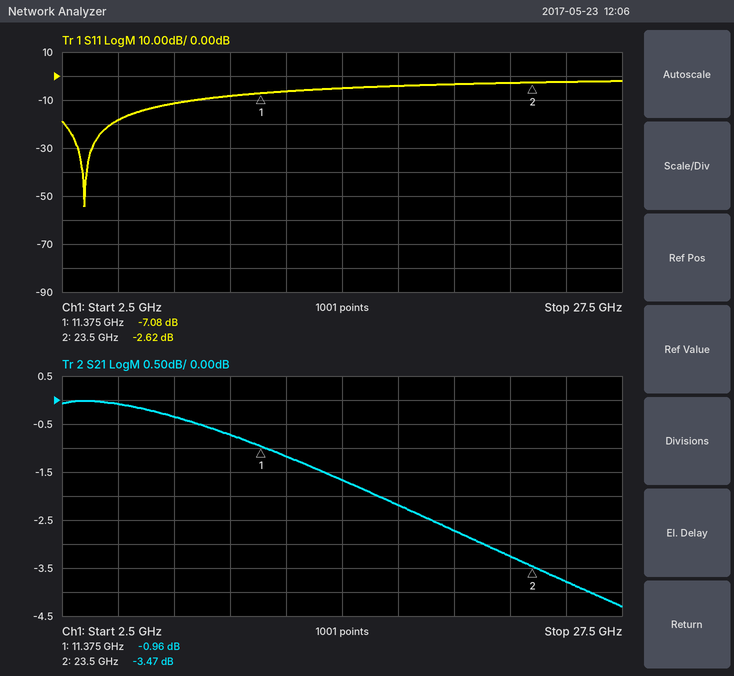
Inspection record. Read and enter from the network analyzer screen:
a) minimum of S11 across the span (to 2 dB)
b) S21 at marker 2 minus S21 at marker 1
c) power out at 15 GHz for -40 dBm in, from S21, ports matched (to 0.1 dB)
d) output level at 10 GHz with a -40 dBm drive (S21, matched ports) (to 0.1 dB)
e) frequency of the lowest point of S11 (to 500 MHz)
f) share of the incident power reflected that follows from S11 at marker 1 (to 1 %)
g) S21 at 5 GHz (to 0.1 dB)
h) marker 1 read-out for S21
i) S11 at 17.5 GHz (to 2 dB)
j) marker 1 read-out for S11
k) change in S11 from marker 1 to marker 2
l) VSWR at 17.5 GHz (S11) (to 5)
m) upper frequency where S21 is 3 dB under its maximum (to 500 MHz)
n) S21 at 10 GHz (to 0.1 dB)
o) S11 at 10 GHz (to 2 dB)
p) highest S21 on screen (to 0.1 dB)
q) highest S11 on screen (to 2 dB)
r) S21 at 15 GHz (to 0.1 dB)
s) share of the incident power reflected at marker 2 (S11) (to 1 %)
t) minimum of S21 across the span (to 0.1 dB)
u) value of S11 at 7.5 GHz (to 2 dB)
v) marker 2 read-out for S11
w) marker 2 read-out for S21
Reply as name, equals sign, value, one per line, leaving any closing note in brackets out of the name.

minimum of S11 across the span = -54 dB
S21 at marker 2 minus S21 at marker 1 = -2.51 dB
power out at 15 GHz for -40 dBm in, from S21, ports matched = -41.7 dBm
output level at 10 GHz with a -40 dBm drive (S21, matched ports) = -40.7 dBm
frequency of the lowest point of S11 = 3.5 GHz
share of the incident power reflected that follows from S11 at marker 1 = 20 %
S21 at 5 GHz = -0.1 dB
marker 1 read-out for S21 = -0.96 dB
S11 at 17.5 GHz = -4 dB
marker 1 read-out for S11 = -7.08 dB
change in S11 from marker 1 to marker 2 = 4.46 dB
VSWR at 17.5 GHz (S11) = 5
upper frequency where S21 is 3 dB under its maximum = 21.5 GHz
S21 at 10 GHz = -0.7 dB
S11 at 10 GHz = -8 dB
highest S21 on screen = 0.0 dB
highest S11 on screen = -2 dB
S21 at 15 GHz = -1.7 dB
share of the incident power reflected at marker 2 (S11) = 55 %
minimum of S21 across the span = -4.3 dB
value of S11 at 7.5 GHz = -12 dB
marker 2 read-out for S11 = -2.62 dB
marker 2 read-out for S21 = -3.47 dB
